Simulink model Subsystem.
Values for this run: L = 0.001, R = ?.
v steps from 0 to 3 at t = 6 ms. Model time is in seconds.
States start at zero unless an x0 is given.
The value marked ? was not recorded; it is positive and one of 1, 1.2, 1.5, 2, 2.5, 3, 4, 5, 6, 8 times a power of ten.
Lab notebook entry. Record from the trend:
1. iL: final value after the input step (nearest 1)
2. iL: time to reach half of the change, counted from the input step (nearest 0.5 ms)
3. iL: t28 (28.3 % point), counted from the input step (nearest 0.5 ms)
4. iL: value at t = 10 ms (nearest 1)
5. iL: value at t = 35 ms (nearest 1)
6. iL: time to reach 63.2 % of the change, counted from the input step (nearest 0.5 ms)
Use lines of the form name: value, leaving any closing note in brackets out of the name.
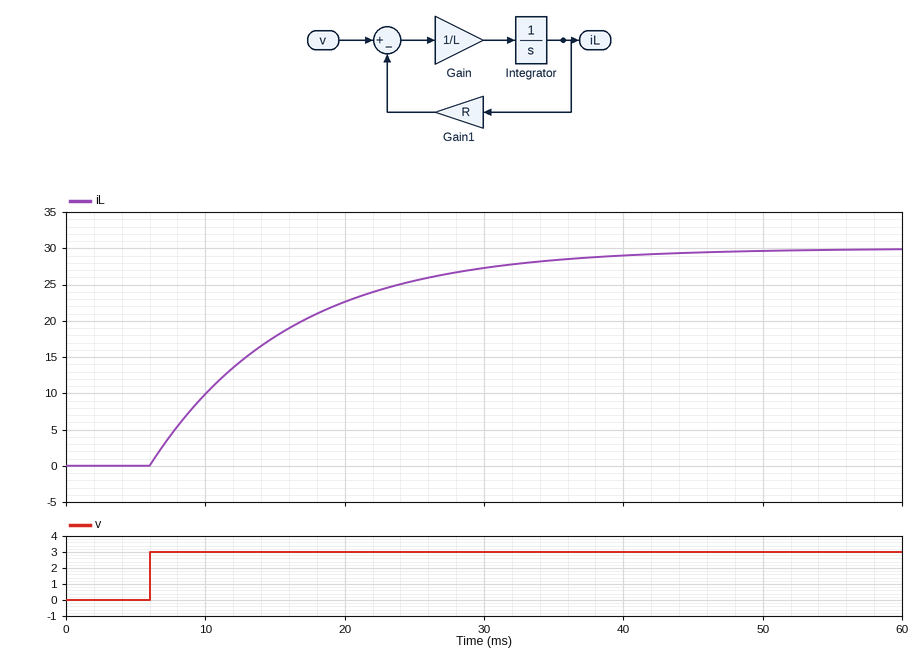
iL: final value after the input step: 30
iL: time to reach half of the change, counted from the input step: 7.0 ms
iL: t28 (28.3 % point), counted from the input step: 3.5 ms
iL: value at t = 10 ms: 10
iL: value at t = 35 ms: 28
iL: time to reach 63.2 % of the change, counted from the input step: 10.0 ms
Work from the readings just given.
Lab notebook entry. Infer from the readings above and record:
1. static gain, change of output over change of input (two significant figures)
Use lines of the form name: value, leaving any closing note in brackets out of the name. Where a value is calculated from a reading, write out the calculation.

static gain, change of output over change of input: (30 - 0) / (3 - 0) = 10
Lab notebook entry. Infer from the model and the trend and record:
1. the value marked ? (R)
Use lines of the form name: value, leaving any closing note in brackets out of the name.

the value marked ?: 0.1
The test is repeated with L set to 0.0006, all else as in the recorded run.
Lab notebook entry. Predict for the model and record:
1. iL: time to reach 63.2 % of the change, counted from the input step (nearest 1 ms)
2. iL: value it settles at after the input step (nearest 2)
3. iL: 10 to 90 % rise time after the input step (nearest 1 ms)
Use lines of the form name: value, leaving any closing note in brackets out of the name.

iL: time to reach 63.2 % of the change, counted from the input step: 6 ms
iL: value it settles at after the input step: 30
iL: 10 to 90 % rise time after the input step: 13 ms
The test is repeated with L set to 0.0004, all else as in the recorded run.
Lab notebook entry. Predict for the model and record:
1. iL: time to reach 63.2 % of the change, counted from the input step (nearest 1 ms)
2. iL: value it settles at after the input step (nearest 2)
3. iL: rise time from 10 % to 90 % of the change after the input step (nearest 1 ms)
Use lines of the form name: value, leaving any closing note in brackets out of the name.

iL: time to reach 63.2 % of the change, counted from the input step: 4 ms
iL: value it settles at after the input step: 30
iL: rise time from 10 % to 90 % of the change after the input step: 9 ms
